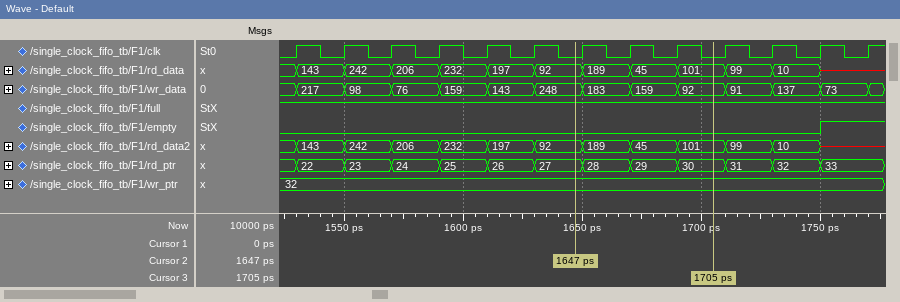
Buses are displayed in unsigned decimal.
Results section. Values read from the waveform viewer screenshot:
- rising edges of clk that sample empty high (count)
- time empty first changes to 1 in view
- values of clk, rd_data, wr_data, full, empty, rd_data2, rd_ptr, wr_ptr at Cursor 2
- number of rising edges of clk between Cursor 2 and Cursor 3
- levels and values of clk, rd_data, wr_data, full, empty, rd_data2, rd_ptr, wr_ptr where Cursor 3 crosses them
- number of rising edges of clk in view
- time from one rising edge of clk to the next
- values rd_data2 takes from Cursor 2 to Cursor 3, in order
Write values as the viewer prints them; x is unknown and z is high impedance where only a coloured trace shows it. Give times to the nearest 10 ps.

1
1750 ps
clk=0, rd_data=92, wr_data=248, full=1, empty=0, rd_data2=92, rd_ptr=27, wr_ptr=32
3
clk=0, rd_data=101, wr_data=92, full=1, empty=0, rd_data2=101, rd_ptr=30, wr_ptr=32
13
20 ps
92, 189, 45, 101
